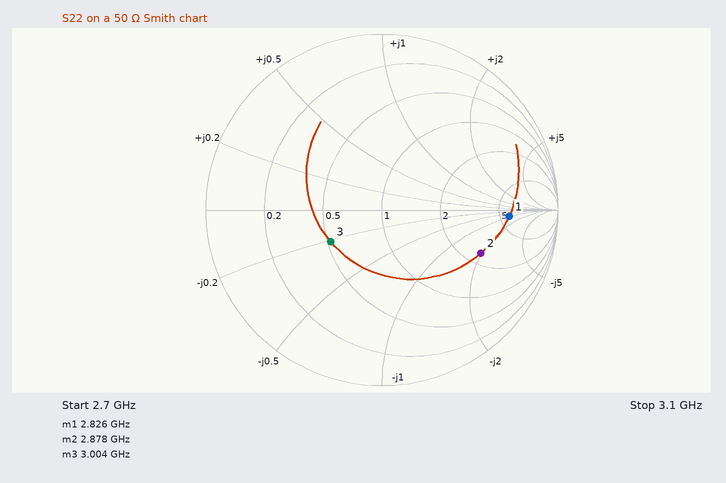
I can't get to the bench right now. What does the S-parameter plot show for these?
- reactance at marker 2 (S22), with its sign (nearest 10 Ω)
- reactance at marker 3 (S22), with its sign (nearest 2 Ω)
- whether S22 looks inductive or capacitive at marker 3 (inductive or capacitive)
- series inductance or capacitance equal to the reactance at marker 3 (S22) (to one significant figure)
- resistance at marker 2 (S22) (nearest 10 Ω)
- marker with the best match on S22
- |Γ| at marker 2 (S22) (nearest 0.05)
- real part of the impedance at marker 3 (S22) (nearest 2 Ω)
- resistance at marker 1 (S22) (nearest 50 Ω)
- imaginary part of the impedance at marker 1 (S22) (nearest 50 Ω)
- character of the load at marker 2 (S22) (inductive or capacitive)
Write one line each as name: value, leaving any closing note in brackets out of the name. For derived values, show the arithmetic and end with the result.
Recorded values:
reactance at marker 2 (S22), with its sign: -100 Ω
reactance at marker 3 (S22), with its sign: -10 Ω
whether S22 looks inductive or capacitive at marker 3: capacitive
series inductance or capacitance equal to the reactance at marker 3 (S22): C = 1/(2π × 3.004 GHz × 10 Ω) ≈ 5 pF
resistance at marker 2 (S22): 120 Ω
marker with the best match on S22: marker 3
|Γ| at marker 2 (S22): 0.60
real part of the impedance at marker 3 (S22): 26 Ω
resistance at marker 1 (S22): 300 Ω
imaginary part of the impedance at marker 1 (S22): -50 Ω
character of the load at marker 2 (S22): capacitive
